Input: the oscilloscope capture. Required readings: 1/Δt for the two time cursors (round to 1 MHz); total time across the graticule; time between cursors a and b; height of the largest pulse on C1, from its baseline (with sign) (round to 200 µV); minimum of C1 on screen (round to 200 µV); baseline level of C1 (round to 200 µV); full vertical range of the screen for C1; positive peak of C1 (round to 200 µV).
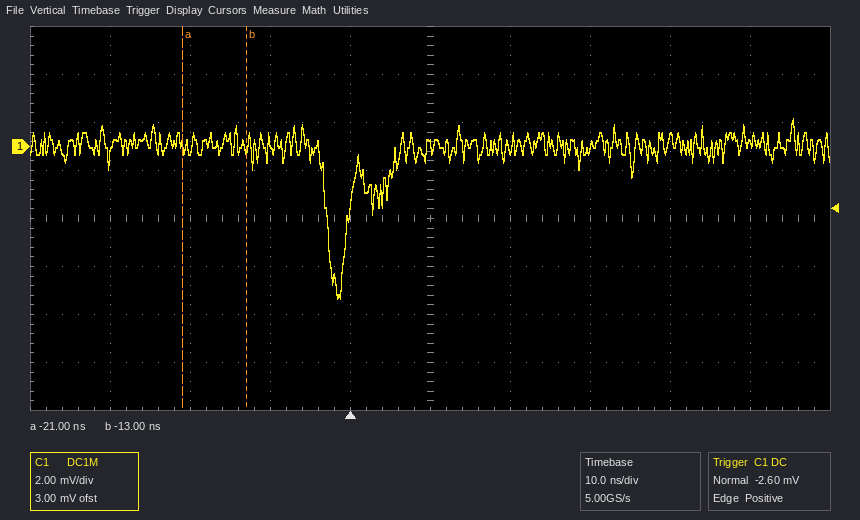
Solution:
125 MHz
100 ns
8 ns
-6.4 mV
-6.4 mV
0.0 mV
16 mV
1.2 mV
